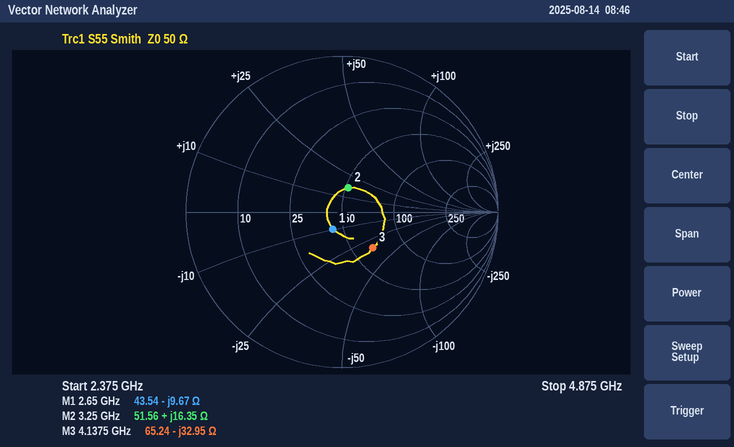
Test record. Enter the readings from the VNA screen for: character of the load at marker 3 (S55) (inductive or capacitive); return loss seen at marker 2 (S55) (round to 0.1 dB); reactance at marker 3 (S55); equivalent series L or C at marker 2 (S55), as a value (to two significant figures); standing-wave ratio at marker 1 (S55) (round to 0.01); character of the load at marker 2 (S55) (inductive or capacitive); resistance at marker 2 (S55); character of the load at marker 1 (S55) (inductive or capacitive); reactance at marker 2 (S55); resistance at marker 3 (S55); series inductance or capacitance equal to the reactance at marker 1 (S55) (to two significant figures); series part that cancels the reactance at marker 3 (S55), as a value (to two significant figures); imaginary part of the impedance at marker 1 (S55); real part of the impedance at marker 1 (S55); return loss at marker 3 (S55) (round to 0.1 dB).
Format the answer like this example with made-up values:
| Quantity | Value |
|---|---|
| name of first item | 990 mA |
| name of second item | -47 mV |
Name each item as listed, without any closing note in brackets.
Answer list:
| Quantity | Value |
|---|---|
| character of the load at marker 3 (S55) | capacitive |
| return loss seen at marker 2 (S55) | 15.9 dB |
| reactance at marker 3 | -32.95 Ω |
| equivalent series L or C at marker 2 (S55), as a value | 800 pH |
| standing-wave ratio at marker 1 (S55) | 1.28 |
| character of the load at marker 2 (S55) | inductive |
| resistance at marker 2 | 51.56 Ω |
| character of the load at marker 1 (S55) | capacitive |
| reactance at marker 2 | +16.35 Ω |
| resistance at marker 3 | 65.24 Ω |
| series inductance or capacitance equal to the reactance at marker 1 (S55) | 6.2 pF |
| series part that cancels the reactance at marker 3 (S55), as a value | 1.3 nH |
| imaginary part of the impedance at marker 1 | -9.67 Ω |
| real part of the impedance at marker 1 | 43.54 Ω |
| return loss at marker 3 (S55) | 10.4 dB |
